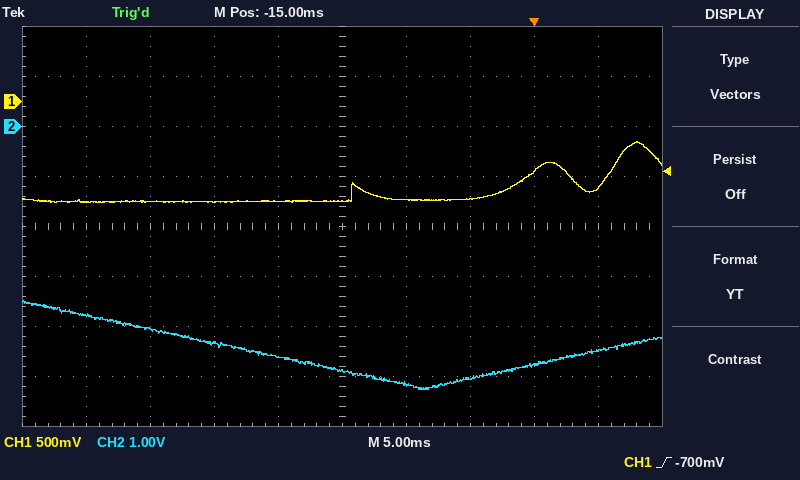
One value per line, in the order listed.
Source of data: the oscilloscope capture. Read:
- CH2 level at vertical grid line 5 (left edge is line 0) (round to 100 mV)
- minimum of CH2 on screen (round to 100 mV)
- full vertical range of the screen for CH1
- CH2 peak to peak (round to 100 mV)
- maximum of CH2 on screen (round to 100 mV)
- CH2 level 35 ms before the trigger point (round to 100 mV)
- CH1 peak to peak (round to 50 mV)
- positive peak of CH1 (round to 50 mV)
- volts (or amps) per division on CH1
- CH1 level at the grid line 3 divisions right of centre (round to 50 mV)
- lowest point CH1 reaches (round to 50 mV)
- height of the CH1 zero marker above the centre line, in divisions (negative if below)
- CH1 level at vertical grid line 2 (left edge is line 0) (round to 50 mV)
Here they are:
-4.9 V
-5.3 V
4 V
1.8 V
-3.5 V
-3.8 V
600 mV
-400 mV
500 mV
-700 mV
-1.00 V
+2.5 div
-1.00 V
